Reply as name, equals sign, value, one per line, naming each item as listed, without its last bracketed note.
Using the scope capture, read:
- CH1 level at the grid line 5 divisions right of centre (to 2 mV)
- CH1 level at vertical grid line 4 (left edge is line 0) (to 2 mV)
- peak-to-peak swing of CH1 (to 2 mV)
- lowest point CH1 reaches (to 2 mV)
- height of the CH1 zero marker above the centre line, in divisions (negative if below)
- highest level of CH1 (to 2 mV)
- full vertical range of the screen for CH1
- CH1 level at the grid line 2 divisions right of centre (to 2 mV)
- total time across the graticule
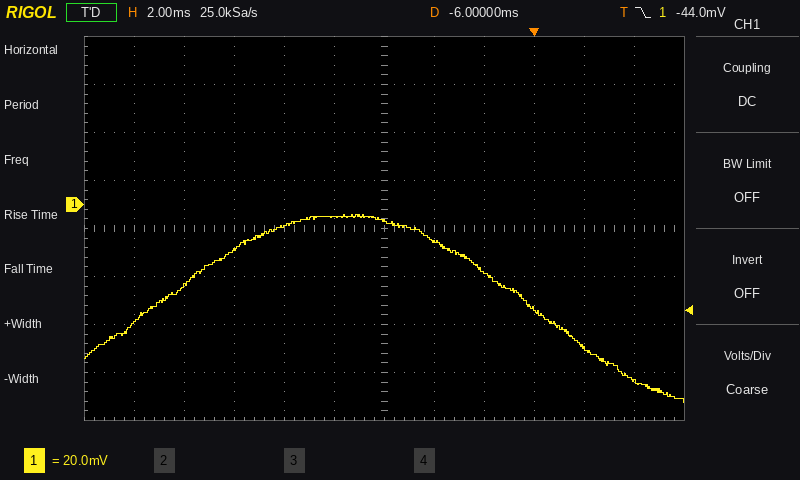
CH1 level at the grid line 5 divisions right of centre = -74 mV
CH1 level at vertical grid line 4 (left edge is line 0) = -8 mV
peak-to-peak swing of CH1 = 78 mV
lowest point CH1 reaches = -82 mV
height of the CH1 zero marker above the centre line, in divisions = +0.5 div
highest level of CH1 = -4 mV
full vertical range of the screen for CH1 = 160 mV
CH1 level at the grid line 2 divisions right of centre = -28 mV
total time across the graticule = 24 ms
